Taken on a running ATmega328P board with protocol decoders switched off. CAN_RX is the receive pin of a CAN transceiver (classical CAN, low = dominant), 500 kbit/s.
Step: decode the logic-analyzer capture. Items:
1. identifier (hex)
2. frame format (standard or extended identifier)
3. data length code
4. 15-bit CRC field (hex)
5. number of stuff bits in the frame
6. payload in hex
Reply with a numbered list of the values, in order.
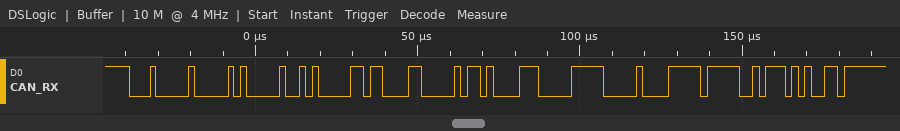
1. 0x100
2. standard
3. 8
4. 0x6BA9
5. 10
6. 0A 0B 0C 0D 0E 0F 00 FF
